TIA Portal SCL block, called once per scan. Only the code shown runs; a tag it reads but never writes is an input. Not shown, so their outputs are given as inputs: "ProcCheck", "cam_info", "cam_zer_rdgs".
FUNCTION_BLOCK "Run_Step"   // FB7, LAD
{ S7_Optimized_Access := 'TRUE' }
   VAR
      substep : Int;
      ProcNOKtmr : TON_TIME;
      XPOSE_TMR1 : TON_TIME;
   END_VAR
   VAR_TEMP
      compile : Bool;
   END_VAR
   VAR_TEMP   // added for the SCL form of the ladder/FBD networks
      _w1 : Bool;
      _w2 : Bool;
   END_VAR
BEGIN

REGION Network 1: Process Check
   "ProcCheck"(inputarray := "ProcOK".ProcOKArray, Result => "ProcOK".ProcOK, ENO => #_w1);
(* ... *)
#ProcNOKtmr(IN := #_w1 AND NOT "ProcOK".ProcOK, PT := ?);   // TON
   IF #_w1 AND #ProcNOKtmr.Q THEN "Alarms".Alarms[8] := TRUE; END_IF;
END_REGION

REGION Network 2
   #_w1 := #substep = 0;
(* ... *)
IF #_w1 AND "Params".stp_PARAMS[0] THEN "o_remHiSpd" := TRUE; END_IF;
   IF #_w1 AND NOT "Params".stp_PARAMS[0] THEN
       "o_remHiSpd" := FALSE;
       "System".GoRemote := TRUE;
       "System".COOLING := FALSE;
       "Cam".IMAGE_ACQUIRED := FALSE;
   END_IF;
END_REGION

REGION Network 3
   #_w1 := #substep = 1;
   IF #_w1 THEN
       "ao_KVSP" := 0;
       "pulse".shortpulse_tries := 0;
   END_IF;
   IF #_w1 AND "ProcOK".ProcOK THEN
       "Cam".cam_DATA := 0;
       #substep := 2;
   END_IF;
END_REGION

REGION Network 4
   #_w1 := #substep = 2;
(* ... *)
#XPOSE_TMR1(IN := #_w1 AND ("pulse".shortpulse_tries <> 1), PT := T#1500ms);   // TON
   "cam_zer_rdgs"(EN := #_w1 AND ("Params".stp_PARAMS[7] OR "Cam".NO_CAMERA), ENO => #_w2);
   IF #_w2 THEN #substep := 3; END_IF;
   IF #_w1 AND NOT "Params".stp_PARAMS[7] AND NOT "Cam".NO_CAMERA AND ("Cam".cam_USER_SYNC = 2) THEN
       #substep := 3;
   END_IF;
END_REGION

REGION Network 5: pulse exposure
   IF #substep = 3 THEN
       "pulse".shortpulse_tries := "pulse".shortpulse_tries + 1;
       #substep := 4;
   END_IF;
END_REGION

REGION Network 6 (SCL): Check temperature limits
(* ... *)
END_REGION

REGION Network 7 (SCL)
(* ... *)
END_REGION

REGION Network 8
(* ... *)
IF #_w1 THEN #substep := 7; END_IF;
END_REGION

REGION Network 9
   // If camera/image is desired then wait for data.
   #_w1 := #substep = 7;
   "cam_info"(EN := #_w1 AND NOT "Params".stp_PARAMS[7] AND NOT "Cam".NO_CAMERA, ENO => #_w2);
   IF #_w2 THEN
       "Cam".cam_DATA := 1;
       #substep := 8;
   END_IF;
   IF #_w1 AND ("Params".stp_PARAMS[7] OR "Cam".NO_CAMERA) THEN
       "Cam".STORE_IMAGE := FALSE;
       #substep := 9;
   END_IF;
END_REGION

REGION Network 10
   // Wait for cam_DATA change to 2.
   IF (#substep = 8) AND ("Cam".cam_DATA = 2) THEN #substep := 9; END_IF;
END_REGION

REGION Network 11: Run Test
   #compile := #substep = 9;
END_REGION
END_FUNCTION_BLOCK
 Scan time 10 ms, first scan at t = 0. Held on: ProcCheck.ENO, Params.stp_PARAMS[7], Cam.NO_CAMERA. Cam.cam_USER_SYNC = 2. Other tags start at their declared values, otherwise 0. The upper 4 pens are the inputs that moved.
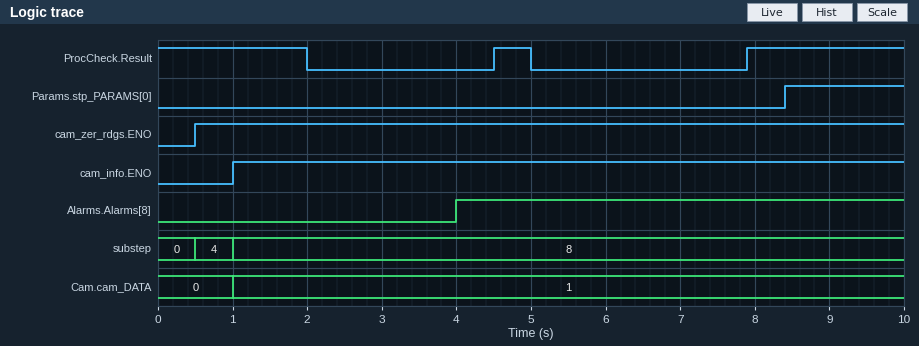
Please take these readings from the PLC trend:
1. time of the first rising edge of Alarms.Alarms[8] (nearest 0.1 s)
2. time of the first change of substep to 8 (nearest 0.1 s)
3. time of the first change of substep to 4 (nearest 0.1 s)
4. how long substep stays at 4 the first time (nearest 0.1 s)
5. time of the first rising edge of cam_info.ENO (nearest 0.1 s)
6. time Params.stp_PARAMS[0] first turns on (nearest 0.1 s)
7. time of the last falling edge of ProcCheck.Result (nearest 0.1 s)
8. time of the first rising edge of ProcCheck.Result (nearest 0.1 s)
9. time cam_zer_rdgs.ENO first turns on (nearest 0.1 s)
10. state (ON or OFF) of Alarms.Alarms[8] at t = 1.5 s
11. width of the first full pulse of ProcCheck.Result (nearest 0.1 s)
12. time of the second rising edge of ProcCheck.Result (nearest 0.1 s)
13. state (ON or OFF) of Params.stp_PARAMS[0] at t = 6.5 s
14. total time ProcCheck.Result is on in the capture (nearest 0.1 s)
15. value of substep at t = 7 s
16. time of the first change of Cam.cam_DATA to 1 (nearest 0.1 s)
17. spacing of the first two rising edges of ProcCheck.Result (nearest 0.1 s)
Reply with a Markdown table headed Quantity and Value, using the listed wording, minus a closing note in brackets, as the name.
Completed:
| Quantity | Value |
|---|---|
| time of the first rising edge of Alarms.Alarms[8] | 4.0 s |
| time of the first change of substep to 8 | 1.0 s |
| time of the first change of substep to 4 | 0.5 s |
| how long substep stays at 4 the first time | 0.5 s |
| time of the first rising edge of cam_info.ENO | 1.0 s |
| time Params.stp_PARAMS[0] first turns on | 8.4 s |
| time of the last falling edge of ProcCheck.Result | 5.0 s |
| time of the first rising edge of ProcCheck.Result | 4.5 s |
| time cam_zer_rdgs.ENO first turns on | 0.5 s |
| state (ON or OFF) of Alarms.Alarms[8] at t = 1.5 s | OFF |
| width of the first full pulse of ProcCheck.Result | 0.5 s |
| time of the second rising edge of ProcCheck.Result | 7.9 s |
| state (ON or OFF) of Params.stp_PARAMS[0] at t = 6.5 s | OFF |
| total time ProcCheck.Result is on in the capture | 4.6 s |
| value of substep at t = 7 s | 8 |
| time of the first change of Cam.cam_DATA to 1 | 1.0 s |
| spacing of the first two rising edges of ProcCheck.Result | 3.4 s |
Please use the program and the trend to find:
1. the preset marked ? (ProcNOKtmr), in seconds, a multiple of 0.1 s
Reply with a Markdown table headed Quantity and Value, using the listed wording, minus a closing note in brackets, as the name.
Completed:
| Quantity | Value |
|---|---|
| the preset marked ? (ProcNOKtmr), in seconds, a multiple of 0.1 s | 2.0 s |
